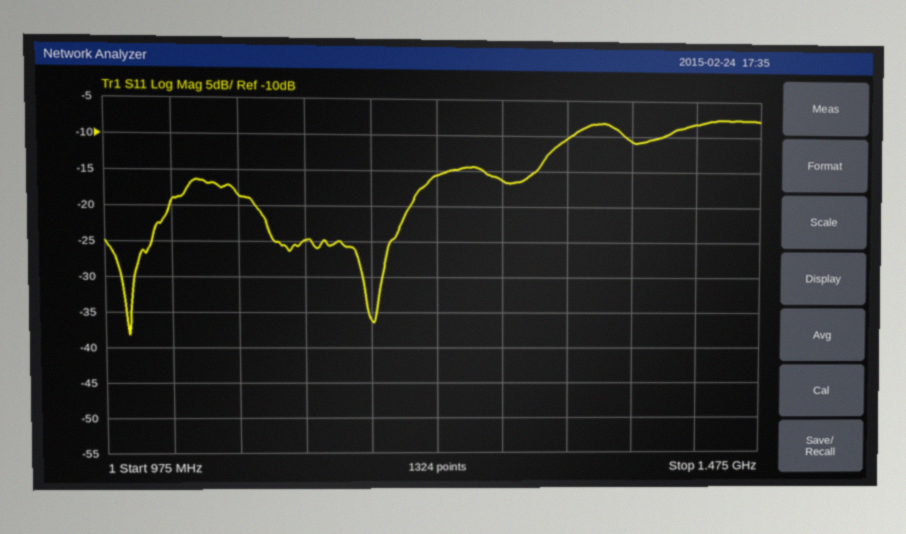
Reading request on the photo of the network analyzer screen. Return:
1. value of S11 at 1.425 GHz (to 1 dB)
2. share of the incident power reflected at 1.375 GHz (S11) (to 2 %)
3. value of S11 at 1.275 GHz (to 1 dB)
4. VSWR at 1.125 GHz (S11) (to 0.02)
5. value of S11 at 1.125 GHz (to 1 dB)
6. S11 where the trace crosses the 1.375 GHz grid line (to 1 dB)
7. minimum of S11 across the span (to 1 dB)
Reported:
-8 dB
8 %
-16 dB
1.12
-25 dB
-11 dB
-38 dB
